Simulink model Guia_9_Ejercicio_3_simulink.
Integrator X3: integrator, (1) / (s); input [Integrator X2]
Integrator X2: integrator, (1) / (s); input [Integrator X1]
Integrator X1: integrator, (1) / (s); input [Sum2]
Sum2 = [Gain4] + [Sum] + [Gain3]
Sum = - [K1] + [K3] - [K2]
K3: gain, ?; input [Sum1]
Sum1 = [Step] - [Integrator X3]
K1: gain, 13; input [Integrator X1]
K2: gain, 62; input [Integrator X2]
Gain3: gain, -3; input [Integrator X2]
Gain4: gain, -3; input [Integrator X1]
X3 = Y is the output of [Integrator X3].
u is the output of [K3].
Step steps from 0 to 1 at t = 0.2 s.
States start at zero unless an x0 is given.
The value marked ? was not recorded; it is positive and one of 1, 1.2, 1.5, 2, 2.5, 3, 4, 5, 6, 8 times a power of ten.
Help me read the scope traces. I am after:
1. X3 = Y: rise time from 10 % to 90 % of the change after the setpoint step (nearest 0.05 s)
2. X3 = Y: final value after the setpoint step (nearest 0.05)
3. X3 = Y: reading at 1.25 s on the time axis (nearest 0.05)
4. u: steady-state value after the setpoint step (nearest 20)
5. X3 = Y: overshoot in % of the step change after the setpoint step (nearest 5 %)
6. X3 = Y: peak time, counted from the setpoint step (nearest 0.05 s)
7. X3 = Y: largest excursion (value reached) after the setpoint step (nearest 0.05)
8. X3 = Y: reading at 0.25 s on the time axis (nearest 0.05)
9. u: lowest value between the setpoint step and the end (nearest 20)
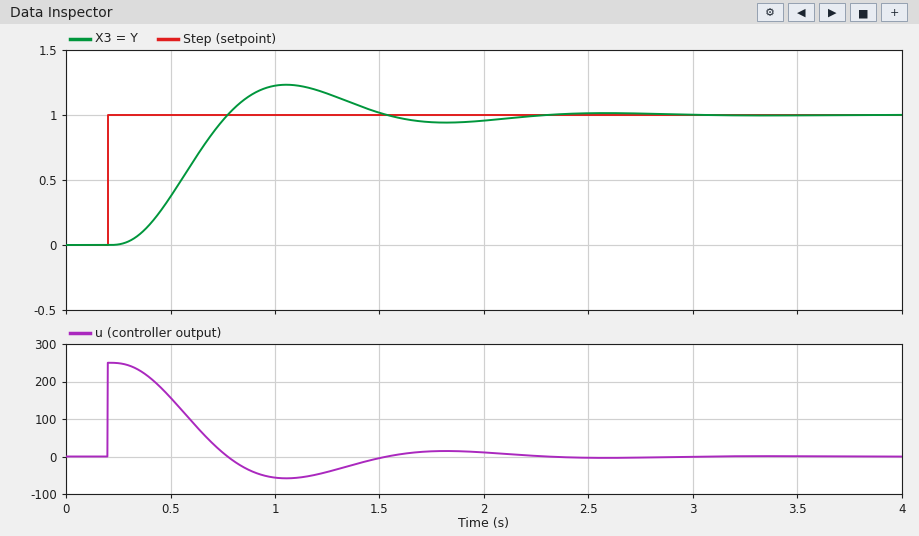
0.35 s
1.00
1.15
0
25 %
0.85 s
1.25
0.00
-60
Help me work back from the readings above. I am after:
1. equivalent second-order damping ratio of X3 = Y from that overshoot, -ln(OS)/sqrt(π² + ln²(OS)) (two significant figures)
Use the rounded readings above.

0.40
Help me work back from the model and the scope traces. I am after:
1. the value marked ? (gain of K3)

250
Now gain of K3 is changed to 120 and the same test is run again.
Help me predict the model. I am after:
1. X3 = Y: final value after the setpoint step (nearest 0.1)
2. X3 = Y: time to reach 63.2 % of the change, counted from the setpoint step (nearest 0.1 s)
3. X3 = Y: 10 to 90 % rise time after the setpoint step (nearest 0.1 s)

1.0
0.6 s
0.7 s
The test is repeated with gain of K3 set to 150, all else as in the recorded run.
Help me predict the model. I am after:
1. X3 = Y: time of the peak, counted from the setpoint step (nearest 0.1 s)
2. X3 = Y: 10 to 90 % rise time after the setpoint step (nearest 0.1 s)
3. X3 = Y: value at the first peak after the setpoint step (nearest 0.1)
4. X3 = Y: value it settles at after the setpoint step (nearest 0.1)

1.2 s
0.6 s
1.1
1.0
